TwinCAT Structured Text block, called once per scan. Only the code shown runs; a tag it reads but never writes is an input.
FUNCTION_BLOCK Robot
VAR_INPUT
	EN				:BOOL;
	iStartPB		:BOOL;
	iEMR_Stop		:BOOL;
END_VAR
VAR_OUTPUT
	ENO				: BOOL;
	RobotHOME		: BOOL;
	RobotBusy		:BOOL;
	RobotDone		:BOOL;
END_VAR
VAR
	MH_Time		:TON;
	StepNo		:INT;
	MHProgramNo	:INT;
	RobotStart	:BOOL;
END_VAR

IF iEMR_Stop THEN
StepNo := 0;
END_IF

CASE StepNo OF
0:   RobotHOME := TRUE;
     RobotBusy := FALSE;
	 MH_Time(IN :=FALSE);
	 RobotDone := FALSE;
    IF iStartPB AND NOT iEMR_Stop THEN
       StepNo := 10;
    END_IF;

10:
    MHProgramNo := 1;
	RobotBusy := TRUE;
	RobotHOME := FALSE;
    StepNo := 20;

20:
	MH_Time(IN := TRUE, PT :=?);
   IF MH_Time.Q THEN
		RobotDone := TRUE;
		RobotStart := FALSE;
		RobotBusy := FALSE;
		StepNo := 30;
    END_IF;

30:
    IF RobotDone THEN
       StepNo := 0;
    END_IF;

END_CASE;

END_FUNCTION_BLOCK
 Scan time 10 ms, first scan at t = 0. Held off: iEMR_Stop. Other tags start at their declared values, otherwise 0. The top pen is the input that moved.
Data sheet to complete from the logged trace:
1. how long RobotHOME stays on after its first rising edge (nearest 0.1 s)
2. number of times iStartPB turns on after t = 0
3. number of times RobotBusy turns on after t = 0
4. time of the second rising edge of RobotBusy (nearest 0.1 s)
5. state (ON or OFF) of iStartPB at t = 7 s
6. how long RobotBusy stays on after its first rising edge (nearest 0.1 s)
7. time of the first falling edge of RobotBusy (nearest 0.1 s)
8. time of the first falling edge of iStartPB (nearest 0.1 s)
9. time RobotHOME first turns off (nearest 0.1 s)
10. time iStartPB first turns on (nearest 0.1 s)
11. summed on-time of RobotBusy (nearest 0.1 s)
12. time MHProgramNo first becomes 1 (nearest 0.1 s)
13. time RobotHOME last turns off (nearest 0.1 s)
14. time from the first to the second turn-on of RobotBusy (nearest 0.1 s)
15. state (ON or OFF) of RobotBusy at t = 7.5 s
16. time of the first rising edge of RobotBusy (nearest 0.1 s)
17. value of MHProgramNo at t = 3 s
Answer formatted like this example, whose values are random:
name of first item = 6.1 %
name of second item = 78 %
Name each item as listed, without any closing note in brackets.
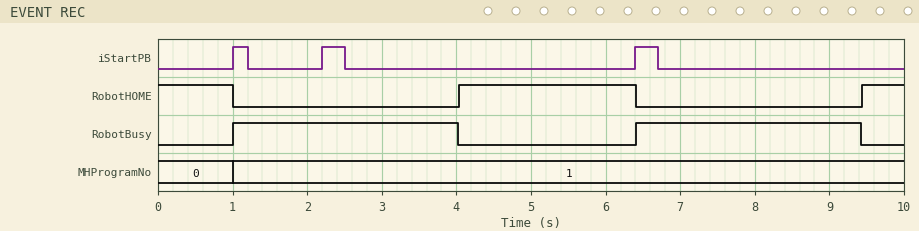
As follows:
how long RobotHOME stays on after its first rising edge = 2.4 s
number of times iStartPB turns on after t = 0 = 3
number of times RobotBusy turns on after t = 0 = 2
time of the second rising edge of RobotBusy = 6.4 s
state (ON or OFF) of iStartPB at t = 7 s = OFF
how long RobotBusy stays on after its first rising edge = 3.0 s
time of the first falling edge of RobotBusy = 4.0 s
time of the first falling edge of iStartPB = 1.2 s
time RobotHOME first turns off = 1.0 s
time iStartPB first turns on = 1.0 s
summed on-time of RobotBusy = 6.0 s
time MHProgramNo first becomes 1 = 1.0 s
time RobotHOME last turns off = 6.4 s
time from the first to the second turn-on of RobotBusy = 5.4 s
state (ON or OFF) of RobotBusy at t = 7.5 s = ON
time of the first rising edge of RobotBusy = 1.0 s
value of MHProgramNo at t = 3 s = 1
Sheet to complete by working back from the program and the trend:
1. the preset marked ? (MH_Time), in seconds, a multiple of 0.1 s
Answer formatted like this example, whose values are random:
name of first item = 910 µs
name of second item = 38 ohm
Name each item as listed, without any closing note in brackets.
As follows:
the preset marked ? (MH_Time), in seconds, a multiple of 0.1 s = 3.0 s
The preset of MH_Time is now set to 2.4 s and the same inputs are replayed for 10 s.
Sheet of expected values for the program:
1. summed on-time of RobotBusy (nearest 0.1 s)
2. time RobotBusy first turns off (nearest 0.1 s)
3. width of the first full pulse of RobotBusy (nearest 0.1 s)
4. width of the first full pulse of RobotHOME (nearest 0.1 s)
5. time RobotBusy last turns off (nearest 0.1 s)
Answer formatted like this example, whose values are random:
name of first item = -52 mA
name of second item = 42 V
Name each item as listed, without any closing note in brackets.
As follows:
summed on-time of RobotBusy = 4.8 s
time RobotBusy first turns off = 3.4 s
width of the first full pulse of RobotBusy = 2.4 s
width of the first full pulse of RobotHOME = 3.0 s
time RobotBusy last turns off = 8.8 s
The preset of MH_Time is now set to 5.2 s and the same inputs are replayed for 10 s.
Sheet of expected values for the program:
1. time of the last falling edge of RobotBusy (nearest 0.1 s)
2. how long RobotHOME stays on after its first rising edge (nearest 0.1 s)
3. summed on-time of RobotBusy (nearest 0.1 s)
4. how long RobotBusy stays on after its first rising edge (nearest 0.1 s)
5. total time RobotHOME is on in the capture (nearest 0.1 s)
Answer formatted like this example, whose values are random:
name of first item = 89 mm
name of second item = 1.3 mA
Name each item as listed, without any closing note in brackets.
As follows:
time of the last falling edge of RobotBusy = 6.2 s
how long RobotHOME stays on after its first rising edge = 0.2 s
summed on-time of RobotBusy = 8.8 s
how long RobotBusy stays on after its first rising edge = 5.2 s
total time RobotHOME is on in the capture = 1.2 s
